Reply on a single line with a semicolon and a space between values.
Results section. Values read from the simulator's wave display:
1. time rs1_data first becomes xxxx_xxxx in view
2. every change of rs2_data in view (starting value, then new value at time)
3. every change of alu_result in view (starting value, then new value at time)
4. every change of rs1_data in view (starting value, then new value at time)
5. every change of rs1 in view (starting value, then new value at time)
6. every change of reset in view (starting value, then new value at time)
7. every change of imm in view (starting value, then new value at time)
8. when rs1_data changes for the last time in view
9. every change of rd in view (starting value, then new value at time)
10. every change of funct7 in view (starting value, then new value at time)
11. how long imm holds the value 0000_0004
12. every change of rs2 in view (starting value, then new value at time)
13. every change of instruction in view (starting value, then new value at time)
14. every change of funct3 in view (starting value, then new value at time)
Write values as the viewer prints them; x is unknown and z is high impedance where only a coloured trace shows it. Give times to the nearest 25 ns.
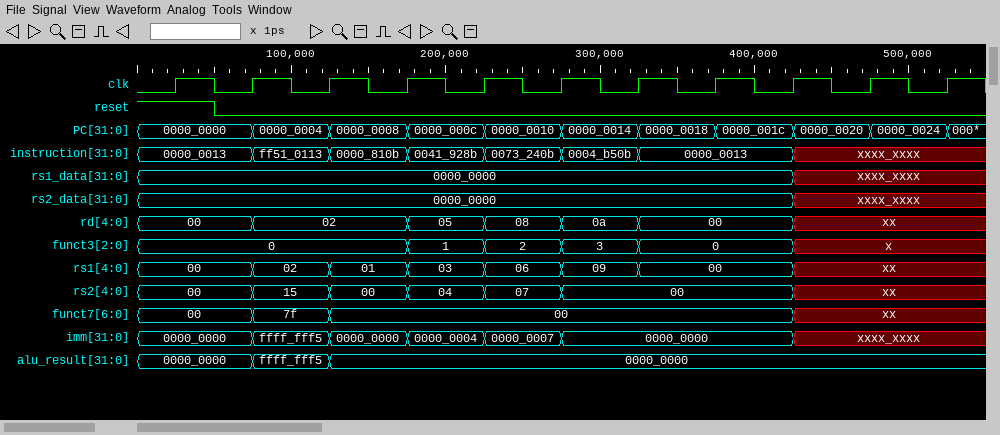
425 ns; 0000_0000, xxxx_xxxx at 425 ns; 0000_0000, ffff_fff5 at 75 ns, 0000_0000 at 125 ns; 0000_0000, xxxx_xxxx at 425 ns; 00, 02 at 75 ns, 01 at 125 ns, 03 at 175 ns, 06 at 225 ns, 09 at 275 ns, 00 at 325 ns, xx at 425 ns; 1, 0 at 50 ns; 0000_0000, ffff_fff5 at 75 ns, 0000_0000 at 125 ns, 0000_0004 at 175 ns, 0000_0007 at 225 ns, 0000_0000 at 275 ns, xxxx_xxxx at 425 ns; 425 ns; 00, 02 at 75 ns, 05 at 175 ns, 08 at 225 ns, 0a at 275 ns, 00 at 325 ns, xx at 425 ns; 00, 7f at 75 ns, 00 at 125 ns, xx at 425 ns; 50 ns; 00, 15 at 75 ns, 00 at 125 ns, 04 at 175 ns, 07 at 225 ns, 00 at 275 ns, xx at 425 ns; 0000_0013, ff51_0113 at 75 ns, 0000_810b at 125 ns, 0041_928b at 175 ns, 0073_240b at 225 ns, 0004_b50b at 275 ns, 0000_0013 at 325 ns, xxxx_xxxx at 425 ns; 0, 1 at 175 ns, 2 at 225 ns, 3 at 275 ns, 0 at 325 ns, x at 425 ns
